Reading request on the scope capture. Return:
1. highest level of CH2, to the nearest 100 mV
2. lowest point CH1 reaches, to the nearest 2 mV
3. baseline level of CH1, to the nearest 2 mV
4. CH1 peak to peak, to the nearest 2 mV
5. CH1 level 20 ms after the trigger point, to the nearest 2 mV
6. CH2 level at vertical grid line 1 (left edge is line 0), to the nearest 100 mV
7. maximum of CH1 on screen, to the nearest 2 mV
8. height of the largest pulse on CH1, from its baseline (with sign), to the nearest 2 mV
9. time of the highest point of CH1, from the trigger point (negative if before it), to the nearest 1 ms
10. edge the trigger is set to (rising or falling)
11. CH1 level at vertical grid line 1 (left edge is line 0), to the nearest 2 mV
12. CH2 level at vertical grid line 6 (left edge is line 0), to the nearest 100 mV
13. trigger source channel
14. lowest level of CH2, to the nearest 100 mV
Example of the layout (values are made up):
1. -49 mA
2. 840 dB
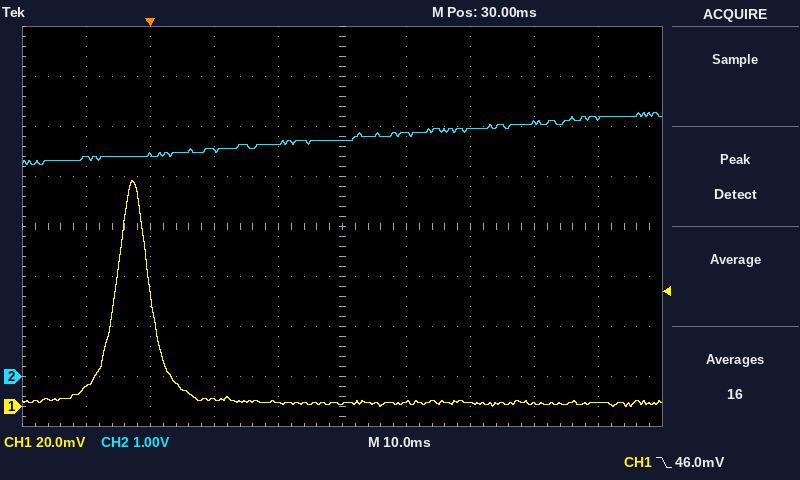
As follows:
1. 5.3 V
2. 0 mV
3. 2 mV
4. 90 mV
5. 2 mV
6. 4.4 V
7. 90 mV
8. +88 mV
9. -3 ms
10. falling
11. 8 mV
12. 4.9 V
13. CH1
14. 4.2 V
